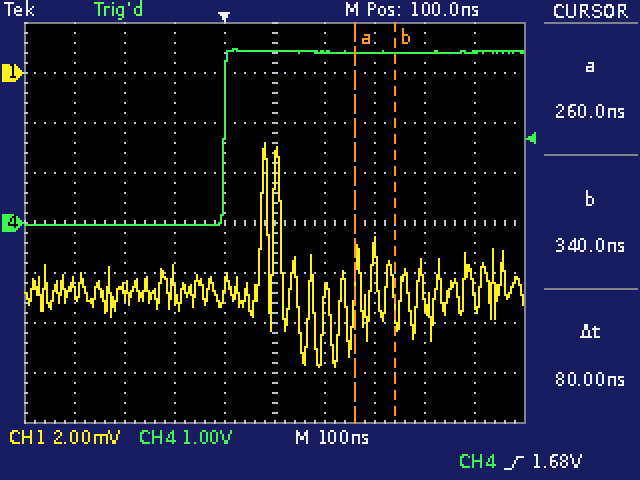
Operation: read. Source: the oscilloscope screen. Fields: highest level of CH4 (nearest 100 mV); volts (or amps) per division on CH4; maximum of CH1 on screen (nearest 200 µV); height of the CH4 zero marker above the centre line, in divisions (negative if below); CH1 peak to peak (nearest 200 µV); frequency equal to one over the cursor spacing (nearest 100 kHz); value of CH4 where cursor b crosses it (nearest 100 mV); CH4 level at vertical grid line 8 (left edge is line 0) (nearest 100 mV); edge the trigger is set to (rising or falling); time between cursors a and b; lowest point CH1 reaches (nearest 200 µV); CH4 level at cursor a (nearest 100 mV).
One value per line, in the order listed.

3.5 V
1 V
-2.8 mV
0.0 div
9.0 mV
12.5 MHz
3.4 V
3.4 V
rising
80 ns
-11.8 mV
3.4 V
